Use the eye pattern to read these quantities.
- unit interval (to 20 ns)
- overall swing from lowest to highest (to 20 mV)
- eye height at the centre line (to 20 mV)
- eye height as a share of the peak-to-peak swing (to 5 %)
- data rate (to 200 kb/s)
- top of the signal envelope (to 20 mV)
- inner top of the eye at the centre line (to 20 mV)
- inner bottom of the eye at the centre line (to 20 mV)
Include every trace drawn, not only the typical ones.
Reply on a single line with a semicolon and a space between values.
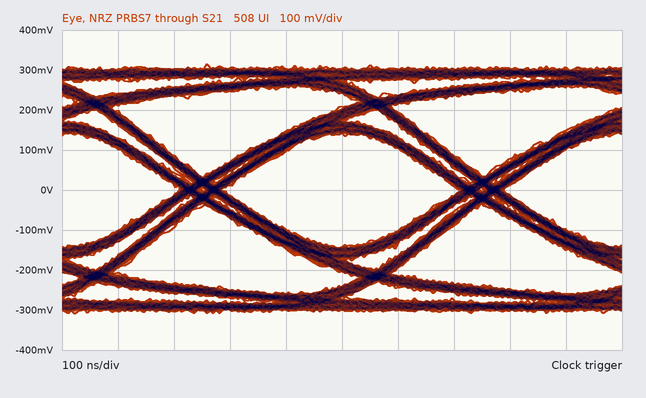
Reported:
500 ns; 620 mV; 280 mV; 45 %; 2.0 Mb/s; 320 mV; 140 mV; -140 mV
